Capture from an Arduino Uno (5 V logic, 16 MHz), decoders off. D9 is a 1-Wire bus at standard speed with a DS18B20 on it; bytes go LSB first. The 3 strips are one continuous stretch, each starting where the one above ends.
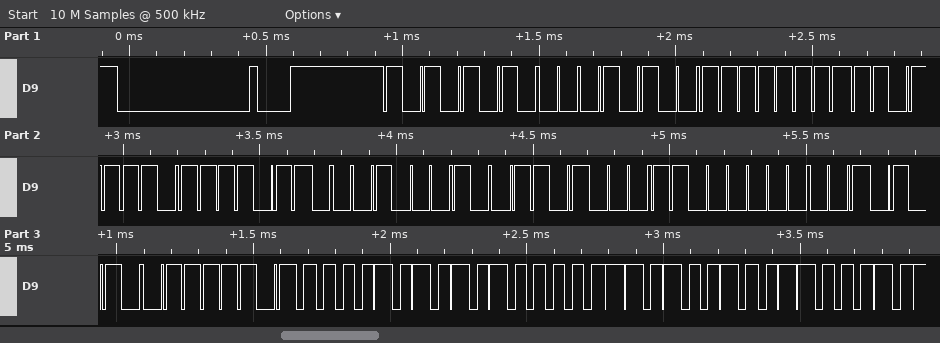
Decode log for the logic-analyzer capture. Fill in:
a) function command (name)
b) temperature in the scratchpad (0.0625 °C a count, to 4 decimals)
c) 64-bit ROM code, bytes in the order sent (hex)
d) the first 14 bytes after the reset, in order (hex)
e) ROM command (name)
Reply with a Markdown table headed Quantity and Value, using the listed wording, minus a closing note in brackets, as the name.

| Quantity | Value |
|---|---|
| function command | Read Scratchpad |
| temperature in the scratchpad | 85.0000 °C |
| 64-bit ROM code, bytes in the order sent | 28 FF 7B 6F 44 16 03 54 |
| the first 14 bytes after the reset, in order | 55 28 FF 7B 6F 44 16 03 54 BE 50 05 4B 46 |
| ROM command | Match ROM |
